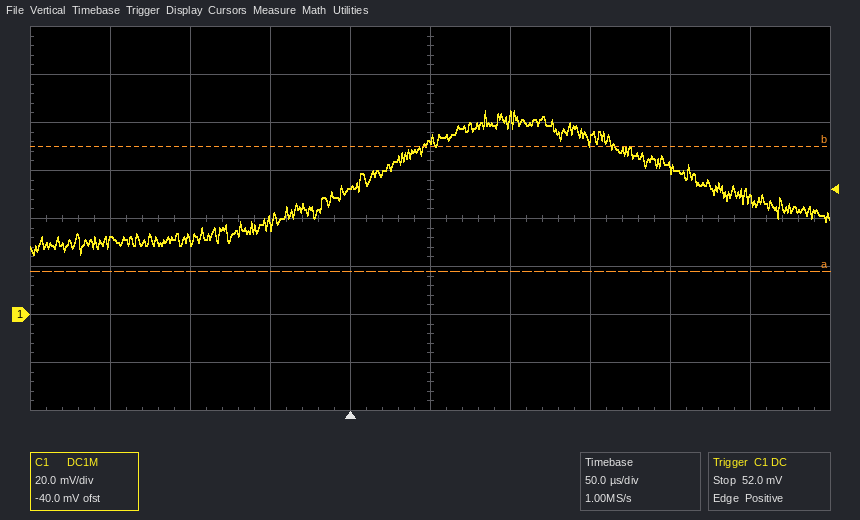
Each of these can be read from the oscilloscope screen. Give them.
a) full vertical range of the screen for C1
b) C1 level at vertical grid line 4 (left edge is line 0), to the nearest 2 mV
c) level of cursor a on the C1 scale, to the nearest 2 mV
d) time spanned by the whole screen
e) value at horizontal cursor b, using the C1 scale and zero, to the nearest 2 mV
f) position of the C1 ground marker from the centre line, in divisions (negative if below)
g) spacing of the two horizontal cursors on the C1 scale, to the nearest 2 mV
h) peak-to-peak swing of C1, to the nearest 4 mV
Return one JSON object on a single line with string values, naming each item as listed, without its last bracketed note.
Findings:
{"full vertical range of the screen for C1": "160 mV", "C1 level at vertical grid line 4 (left edge is line 0), to the nearest 2 mV": "52 mV", "level of cursor a on the C1 scale, to the nearest 2 mV": "18 mV", "time spanned by the whole screen": "500 µs", "value at horizontal cursor b, using the C1 scale and zero, to the nearest 2 mV": "70 mV", "position of the C1 ground marker from the centre line, in divisions": "-2.0 div", "spacing of the two horizontal cursors on the C1 scale, to the nearest 2 mV": "52 mV", "peak-to-peak swing of C1, to the nearest 4 mV": "60 mV"}
